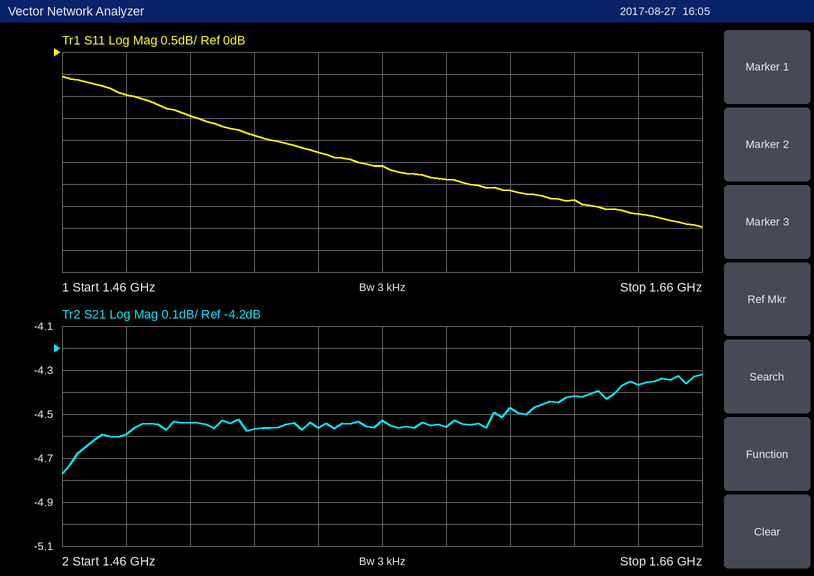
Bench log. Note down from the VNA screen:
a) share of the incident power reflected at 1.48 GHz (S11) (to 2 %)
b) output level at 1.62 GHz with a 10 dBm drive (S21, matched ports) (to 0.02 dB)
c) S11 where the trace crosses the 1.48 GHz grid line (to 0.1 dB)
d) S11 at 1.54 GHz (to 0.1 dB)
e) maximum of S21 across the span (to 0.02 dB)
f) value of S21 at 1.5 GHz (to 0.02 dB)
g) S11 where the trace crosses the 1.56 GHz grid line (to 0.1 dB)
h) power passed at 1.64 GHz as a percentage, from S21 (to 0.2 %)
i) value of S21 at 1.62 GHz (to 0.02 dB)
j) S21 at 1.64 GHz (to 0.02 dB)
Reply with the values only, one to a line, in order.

80 %
5.58 dBm
-1.0 dB
-2.3 dB
-4.32 dB
-4.54 dB
-2.6 dB
36.6 %
-4.42 dB
-4.36 dB
